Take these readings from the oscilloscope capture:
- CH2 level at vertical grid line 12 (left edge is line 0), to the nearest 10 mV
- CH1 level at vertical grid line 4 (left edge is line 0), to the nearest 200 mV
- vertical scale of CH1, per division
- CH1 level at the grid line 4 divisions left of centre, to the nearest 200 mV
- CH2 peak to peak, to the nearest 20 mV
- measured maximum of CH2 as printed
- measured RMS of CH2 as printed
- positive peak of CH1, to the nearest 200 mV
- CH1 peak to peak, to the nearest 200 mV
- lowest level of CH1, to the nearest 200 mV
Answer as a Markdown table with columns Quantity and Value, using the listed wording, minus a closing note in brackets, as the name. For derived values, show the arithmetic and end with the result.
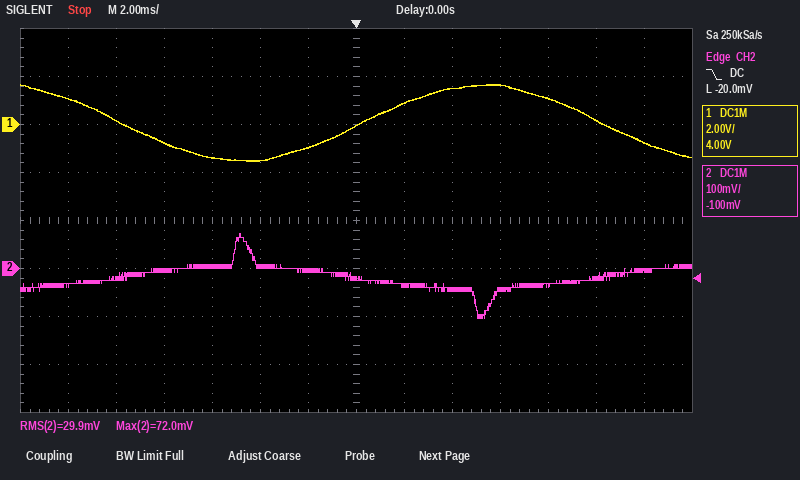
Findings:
| Quantity | Value |
|---|---|
| CH2 level at vertical grid line 12 (left edge is line 0), to the nearest 10 mV | -20 mV |
| CH1 level at vertical grid line 4 (left edge is line 0), to the nearest 200 mV | -1.4 V |
| vertical scale of CH1, per division | 2 V |
| CH1 level at the grid line 4 divisions left of centre, to the nearest 200 mV | -800 mV |
| CH2 peak to peak, to the nearest 20 mV | 180 mV |
| measured maximum of CH2 as printed | 72.0 mV |
| measured RMS of CH2 as printed | 29.9 mV |
| positive peak of CH1, to the nearest 200 mV | 1.6 V |
| CH1 peak to peak, to the nearest 200 mV | 1.6 V − (-1.6 V) = 3.2 V |
| lowest level of CH1, to the nearest 200 mV | -1.6 V |
